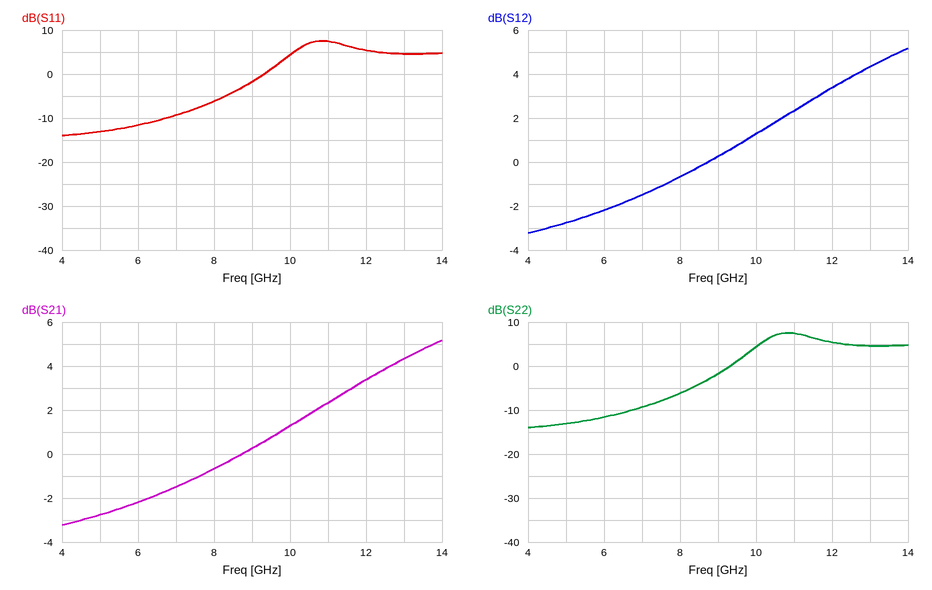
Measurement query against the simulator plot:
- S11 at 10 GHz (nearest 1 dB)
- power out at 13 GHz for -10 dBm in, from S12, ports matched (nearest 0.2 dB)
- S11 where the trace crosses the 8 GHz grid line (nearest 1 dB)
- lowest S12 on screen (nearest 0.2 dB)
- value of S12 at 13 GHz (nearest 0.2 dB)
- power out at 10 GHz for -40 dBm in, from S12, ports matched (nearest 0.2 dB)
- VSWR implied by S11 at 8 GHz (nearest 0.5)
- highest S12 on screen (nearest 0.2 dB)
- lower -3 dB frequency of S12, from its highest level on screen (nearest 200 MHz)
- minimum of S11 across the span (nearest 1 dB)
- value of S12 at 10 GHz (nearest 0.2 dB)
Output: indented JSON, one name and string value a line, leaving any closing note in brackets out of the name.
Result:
{
  "S11 at 10 GHz": "4 dB",
  "power out at 13 GHz for -10 dBm in, from S12, ports matched": "-5.6 dBm",
  "S11 where the trace crosses the 8 GHz grid line": "-6 dB",
  "lowest S12 on screen": "-3.2 dB",
  "value of S12 at 13 GHz": "4.4 dB",
  "power out at 10 GHz for -40 dBm in, from S12, ports matched": "-38.8 dBm",
  "VSWR implied by S11 at 8 GHz": "3.0",
  "highest S12 on screen": "5.2 dB",
  "lower -3 dB frequency of S12, from its highest level on screen": "10.8 GHz",
  "minimum of S11 across the span": "-14 dB",
  "value of S12 at 10 GHz": "1.2 dB"
}
